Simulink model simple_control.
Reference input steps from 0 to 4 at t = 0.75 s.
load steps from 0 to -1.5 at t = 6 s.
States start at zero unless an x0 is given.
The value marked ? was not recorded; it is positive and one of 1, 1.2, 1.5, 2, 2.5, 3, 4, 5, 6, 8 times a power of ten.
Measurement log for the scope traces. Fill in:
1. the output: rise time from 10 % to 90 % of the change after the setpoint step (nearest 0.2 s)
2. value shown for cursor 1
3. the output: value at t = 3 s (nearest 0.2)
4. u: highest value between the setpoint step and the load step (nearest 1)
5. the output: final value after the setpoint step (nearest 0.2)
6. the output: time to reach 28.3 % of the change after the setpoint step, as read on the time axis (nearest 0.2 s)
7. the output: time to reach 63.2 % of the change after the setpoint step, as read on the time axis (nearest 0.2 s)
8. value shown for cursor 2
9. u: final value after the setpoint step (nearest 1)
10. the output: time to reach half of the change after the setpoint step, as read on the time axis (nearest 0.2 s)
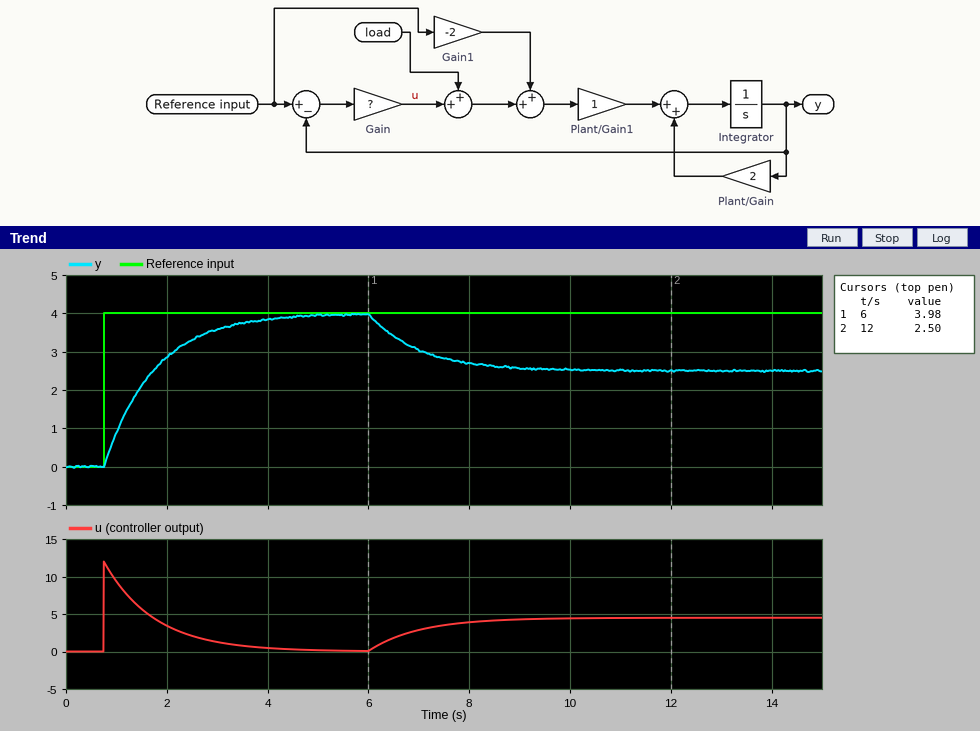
2.2 s
3.98
3.6
12
4.0
1.0 s
1.8 s
2.50
0
1.4 s
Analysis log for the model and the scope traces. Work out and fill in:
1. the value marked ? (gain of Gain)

3
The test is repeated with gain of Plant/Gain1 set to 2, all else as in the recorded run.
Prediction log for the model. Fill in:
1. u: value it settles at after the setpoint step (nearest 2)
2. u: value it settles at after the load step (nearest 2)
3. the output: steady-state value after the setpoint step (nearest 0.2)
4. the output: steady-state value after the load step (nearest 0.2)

6
8
2.0
1.2
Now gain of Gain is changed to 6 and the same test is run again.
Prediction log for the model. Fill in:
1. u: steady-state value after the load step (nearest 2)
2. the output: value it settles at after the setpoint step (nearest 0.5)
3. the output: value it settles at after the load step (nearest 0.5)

2
4.0
3.5
